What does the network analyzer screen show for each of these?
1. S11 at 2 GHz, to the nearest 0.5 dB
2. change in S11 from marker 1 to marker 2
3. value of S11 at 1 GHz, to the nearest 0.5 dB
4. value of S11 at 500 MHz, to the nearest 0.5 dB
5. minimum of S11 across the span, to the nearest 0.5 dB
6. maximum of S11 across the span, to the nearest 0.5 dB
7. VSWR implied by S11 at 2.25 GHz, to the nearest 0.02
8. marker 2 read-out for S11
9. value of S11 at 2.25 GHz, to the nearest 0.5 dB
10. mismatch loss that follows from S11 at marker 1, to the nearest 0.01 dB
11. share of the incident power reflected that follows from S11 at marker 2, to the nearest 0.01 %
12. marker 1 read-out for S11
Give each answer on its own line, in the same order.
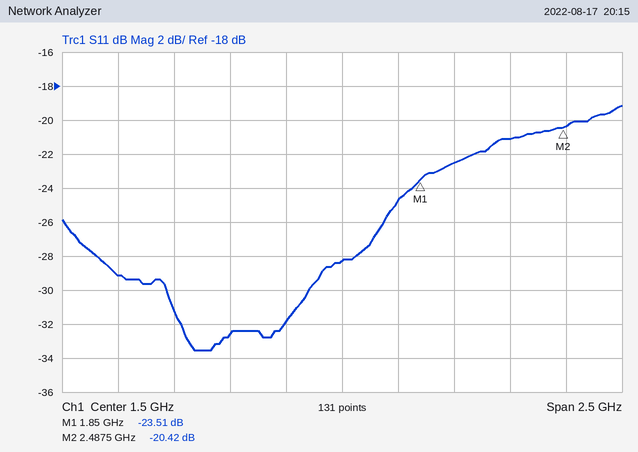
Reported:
-22.5 dB
3.09 dB
-32.5 dB
-29.0 dB
-33.5 dB
-19.0 dB
1.20
-20.42 dB
-21.0 dB
0.02 dB
0.91 %
-23.51 dB
